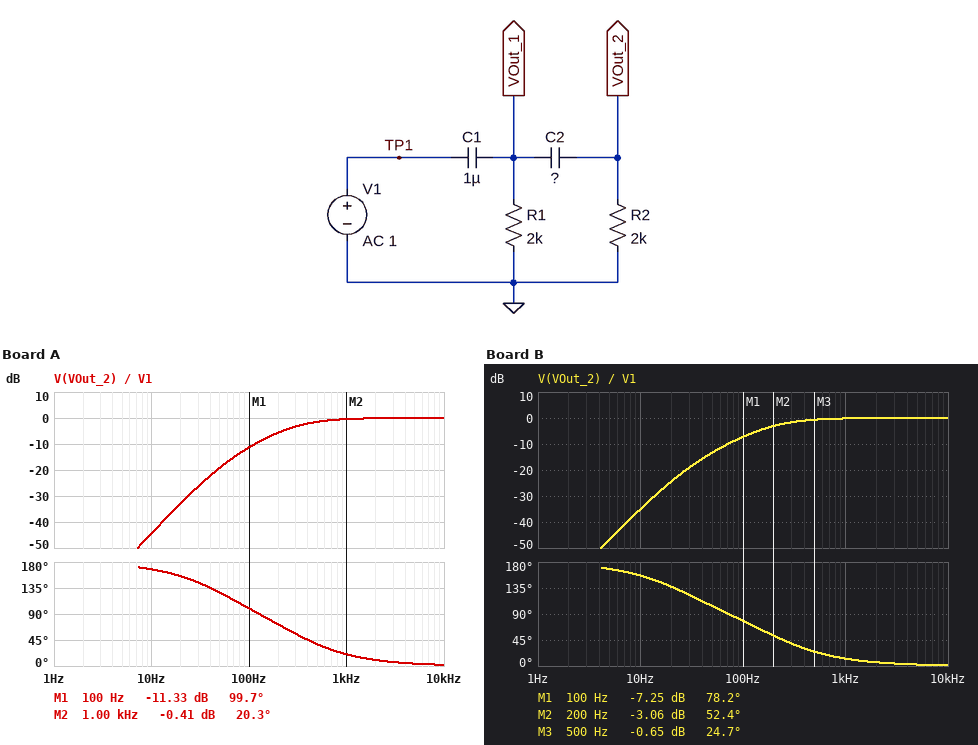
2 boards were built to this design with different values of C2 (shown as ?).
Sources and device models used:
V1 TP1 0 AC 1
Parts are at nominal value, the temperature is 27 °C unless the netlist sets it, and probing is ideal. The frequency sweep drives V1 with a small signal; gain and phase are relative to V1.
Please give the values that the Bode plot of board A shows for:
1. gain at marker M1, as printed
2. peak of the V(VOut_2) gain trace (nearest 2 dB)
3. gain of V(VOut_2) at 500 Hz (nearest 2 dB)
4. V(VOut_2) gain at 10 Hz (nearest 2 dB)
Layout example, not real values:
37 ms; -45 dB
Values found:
-11.33 dB; 0 dB; -2 dB; -44 dB
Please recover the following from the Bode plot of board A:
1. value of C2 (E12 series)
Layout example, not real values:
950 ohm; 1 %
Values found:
390 nF
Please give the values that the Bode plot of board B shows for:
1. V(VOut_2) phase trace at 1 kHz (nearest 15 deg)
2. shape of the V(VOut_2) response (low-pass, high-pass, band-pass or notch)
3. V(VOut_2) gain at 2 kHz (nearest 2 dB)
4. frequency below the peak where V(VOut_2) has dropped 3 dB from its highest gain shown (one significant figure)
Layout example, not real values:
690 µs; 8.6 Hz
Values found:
15 deg; high-pass; 0 dB; 200 Hz
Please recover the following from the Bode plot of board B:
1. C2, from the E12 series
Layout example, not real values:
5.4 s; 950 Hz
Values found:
1.2 µF
